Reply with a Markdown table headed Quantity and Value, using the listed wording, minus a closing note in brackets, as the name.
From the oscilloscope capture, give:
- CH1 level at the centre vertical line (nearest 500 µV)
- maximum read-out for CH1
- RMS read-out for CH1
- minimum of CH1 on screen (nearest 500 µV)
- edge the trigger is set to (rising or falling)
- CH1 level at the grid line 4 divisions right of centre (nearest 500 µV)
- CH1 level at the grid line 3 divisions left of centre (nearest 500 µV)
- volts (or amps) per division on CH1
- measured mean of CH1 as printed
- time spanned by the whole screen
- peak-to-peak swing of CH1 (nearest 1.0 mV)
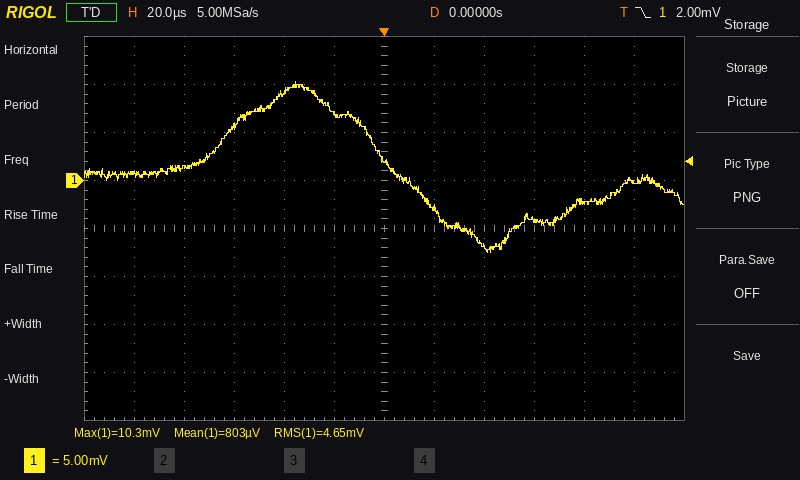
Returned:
| Quantity | Value |
|---|---|
| CH1 level at the centre vertical line | 2.0 mV |
| maximum read-out for CH1 | 10.3 mV |
| RMS read-out for CH1 | 4.65 mV |
| minimum of CH1 on screen | -7.5 mV |
| edge the trigger is set to | falling |
| CH1 level at the grid line 4 divisions right of centre | -2.0 mV |
| CH1 level at the grid line 3 divisions left of centre | 5.5 mV |
| volts (or amps) per division on CH1 | 5 mV |
| measured mean of CH1 as printed | 803 µV |
| time spanned by the whole screen | 240 µs |
| peak-to-peak swing of CH1 | 18.0 mV |
